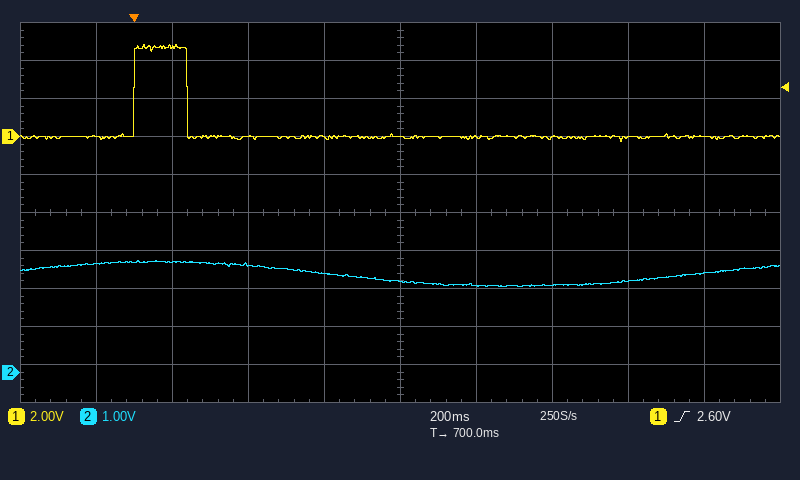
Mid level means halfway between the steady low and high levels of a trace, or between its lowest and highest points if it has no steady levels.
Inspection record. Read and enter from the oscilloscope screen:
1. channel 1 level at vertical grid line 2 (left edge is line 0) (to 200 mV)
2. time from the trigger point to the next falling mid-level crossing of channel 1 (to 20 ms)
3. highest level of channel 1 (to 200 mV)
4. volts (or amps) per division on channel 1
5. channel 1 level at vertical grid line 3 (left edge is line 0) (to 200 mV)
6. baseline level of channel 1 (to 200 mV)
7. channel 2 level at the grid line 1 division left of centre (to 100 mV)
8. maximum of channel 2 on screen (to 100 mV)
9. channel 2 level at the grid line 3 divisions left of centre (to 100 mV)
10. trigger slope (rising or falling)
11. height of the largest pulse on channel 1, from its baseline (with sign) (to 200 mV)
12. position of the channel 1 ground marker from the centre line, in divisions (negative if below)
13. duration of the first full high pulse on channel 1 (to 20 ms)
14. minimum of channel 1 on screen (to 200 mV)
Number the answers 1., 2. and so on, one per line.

1. 4.8 V
2. 140 ms
3. 4.8 V
4. 2 V
5. 0.0 V
6. 0.0 V
7. 2.6 V
8. 2.9 V
9. 2.9 V
10. rising
11. +4.8 V
12. +2.0 div
13. 140 ms
14. -200 mV
